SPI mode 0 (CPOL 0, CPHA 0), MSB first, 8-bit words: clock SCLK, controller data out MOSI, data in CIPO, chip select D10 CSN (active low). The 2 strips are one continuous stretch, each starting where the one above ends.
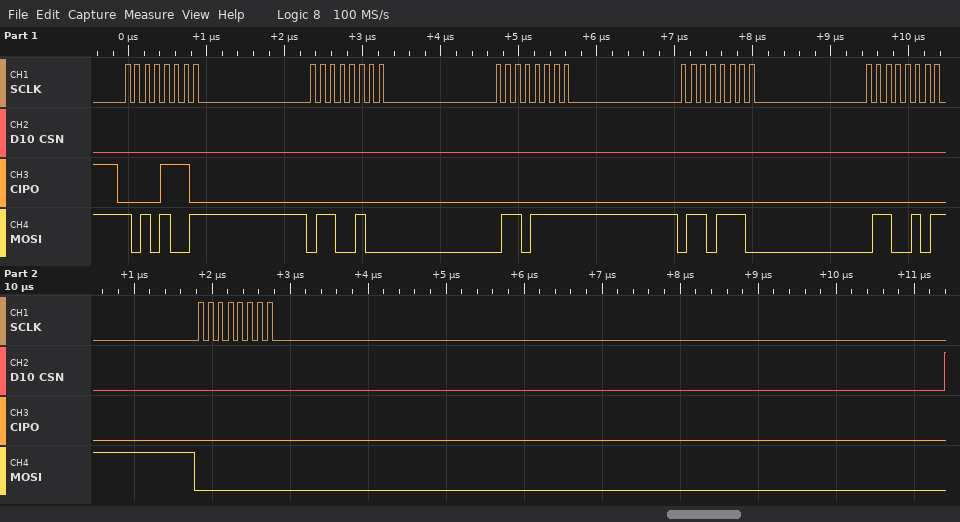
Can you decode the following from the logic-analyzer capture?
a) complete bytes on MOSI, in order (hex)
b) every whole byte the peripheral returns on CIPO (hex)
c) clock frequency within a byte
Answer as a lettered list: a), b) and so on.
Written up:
a) A9 64 6F 6E 65 00
b) 0E 00 00 00 00 00
c) 8 MHz
